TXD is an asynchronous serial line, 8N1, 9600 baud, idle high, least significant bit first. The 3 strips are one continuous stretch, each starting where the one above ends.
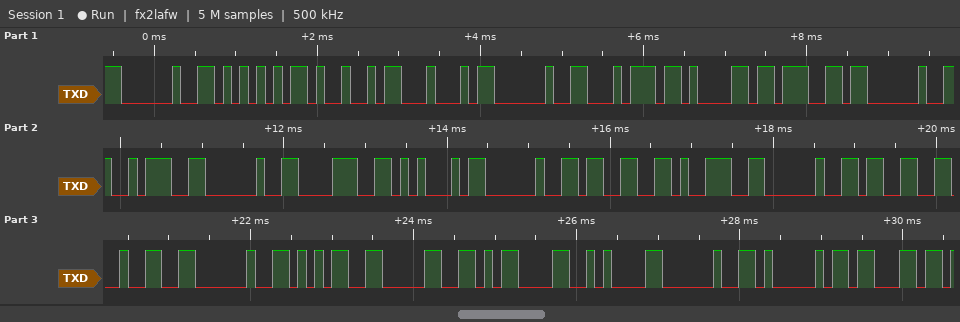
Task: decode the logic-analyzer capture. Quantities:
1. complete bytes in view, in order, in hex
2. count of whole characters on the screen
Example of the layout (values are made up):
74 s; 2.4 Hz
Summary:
20 55 49 44 20 74 61 67 20 3A 20 38 45 20 33 39 20 33 32 20 35 30 0D 0A 20 41 63; 27
